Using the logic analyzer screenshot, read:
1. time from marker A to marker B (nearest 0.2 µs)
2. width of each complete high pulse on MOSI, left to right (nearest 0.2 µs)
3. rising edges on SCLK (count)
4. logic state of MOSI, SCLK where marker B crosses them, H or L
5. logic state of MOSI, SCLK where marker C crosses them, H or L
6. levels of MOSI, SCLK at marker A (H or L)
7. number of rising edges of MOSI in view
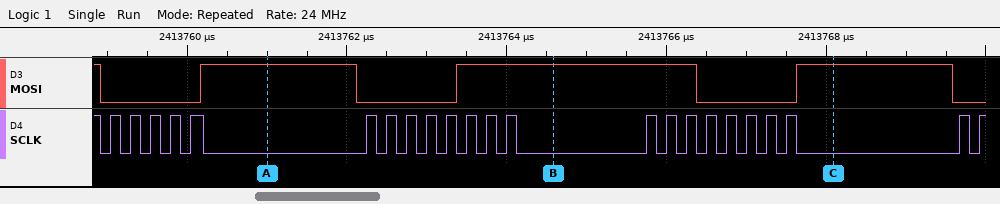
3.6 µs
2 µs, 3 µs, 2 µs
23
MOSI=H, SCLK=L
MOSI=H, SCLK=L
MOSI=H, SCLK=L
3
